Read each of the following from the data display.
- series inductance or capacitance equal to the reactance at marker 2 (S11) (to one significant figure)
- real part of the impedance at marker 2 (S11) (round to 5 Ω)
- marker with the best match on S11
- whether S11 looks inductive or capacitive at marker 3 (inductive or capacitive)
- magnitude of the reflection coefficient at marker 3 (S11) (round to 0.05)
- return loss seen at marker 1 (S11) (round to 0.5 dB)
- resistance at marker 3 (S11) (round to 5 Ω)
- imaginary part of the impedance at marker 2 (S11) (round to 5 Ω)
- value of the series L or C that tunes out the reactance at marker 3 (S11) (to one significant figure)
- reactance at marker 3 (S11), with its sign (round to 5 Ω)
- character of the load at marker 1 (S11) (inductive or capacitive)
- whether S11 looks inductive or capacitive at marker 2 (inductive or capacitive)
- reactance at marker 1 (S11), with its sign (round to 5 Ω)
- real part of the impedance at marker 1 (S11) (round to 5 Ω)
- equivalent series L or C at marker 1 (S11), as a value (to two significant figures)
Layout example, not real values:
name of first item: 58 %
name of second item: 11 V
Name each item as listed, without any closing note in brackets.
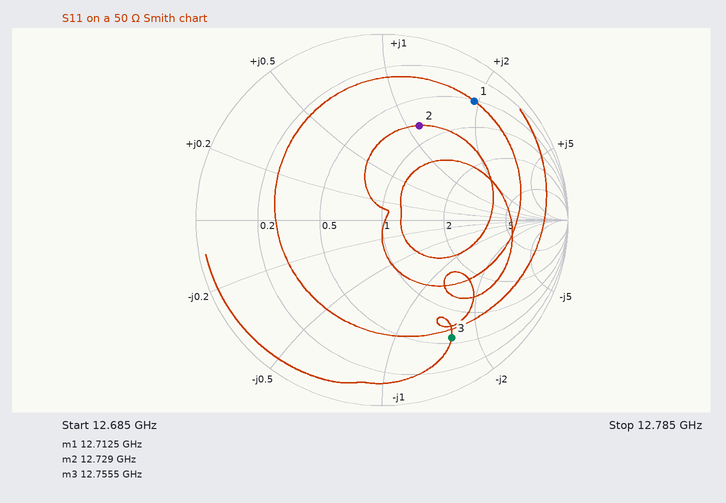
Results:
series inductance or capacitance equal to the reactance at marker 2 (S11): 700 pH
real part of the impedance at marker 2 (S11): 40 Ω
marker with the best match on S11: marker 2
whether S11 looks inductive or capacitive at marker 3: capacitive
magnitude of the reflection coefficient at marker 3 (S11): 0.75
return loss seen at marker 1 (S11): 2.0 dB
resistance at marker 3 (S11): 30 Ω
imaginary part of the impedance at marker 2 (S11): +55 Ω
value of the series L or C that tunes out the reactance at marker 3 (S11): 1.0 nH
reactance at marker 3 (S11), with its sign: -80 Ω
character of the load at marker 1 (S11): inductive
whether S11 looks inductive or capacitive at marker 2: inductive
reactance at marker 1 (S11), with its sign: +95 Ω
real part of the impedance at marker 1 (S11): 25 Ω
equivalent series L or C at marker 1 (S11), as a value: 1.2 nH
